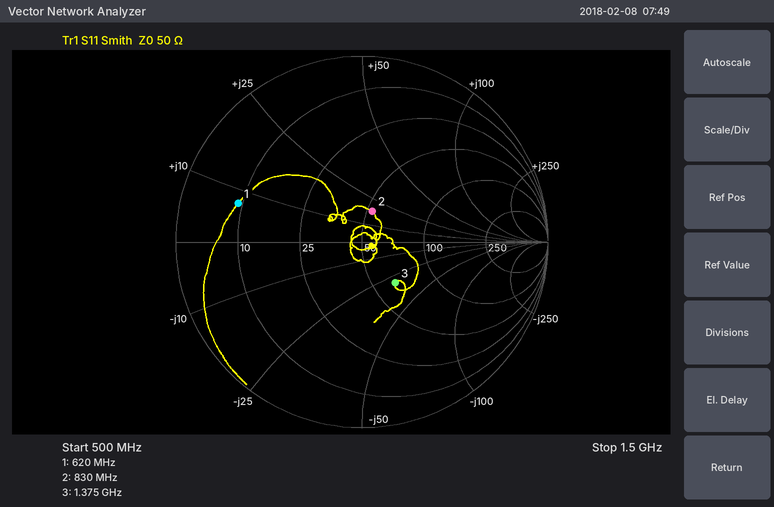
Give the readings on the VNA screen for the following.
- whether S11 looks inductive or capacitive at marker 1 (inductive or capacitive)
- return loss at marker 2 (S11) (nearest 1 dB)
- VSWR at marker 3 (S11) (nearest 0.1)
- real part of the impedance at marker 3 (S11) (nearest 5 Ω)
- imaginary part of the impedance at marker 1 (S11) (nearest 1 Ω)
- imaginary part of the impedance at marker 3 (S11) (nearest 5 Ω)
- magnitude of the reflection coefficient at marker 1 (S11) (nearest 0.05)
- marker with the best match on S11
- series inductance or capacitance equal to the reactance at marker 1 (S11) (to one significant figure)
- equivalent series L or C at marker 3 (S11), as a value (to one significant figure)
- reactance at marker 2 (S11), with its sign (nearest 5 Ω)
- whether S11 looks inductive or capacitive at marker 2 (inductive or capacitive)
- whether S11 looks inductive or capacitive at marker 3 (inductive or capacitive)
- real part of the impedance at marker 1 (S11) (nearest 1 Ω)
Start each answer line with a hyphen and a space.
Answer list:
- inductive
- 15 dB
- 1.8
- 65 Ω
- +7 Ω
- -30 Ω
- 0.70
- marker 2
- 2 nH
- 4 pF
- +20 Ω
- inductive
- capacitive
- 9 Ω
